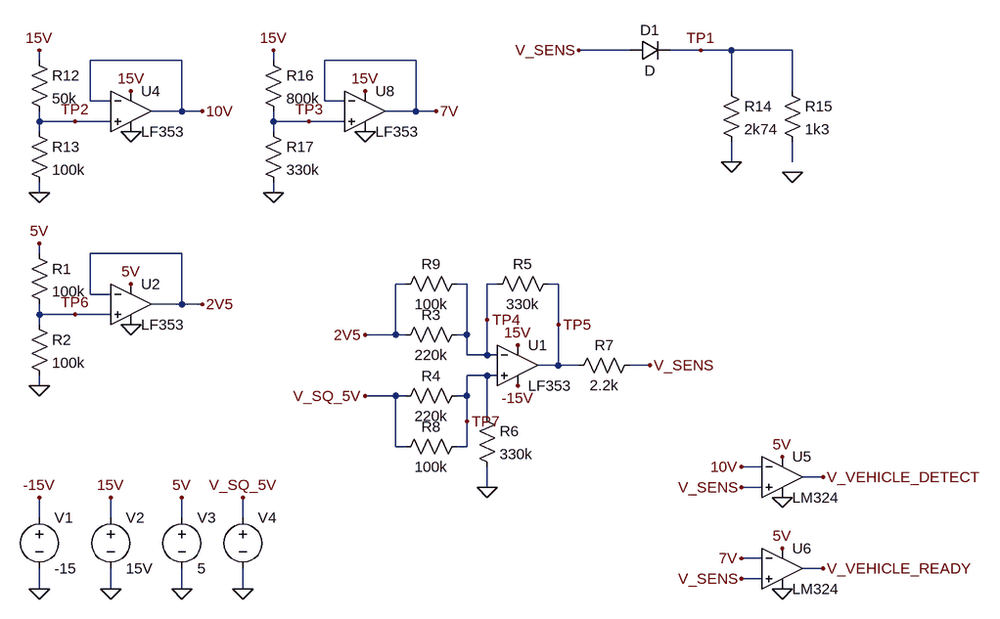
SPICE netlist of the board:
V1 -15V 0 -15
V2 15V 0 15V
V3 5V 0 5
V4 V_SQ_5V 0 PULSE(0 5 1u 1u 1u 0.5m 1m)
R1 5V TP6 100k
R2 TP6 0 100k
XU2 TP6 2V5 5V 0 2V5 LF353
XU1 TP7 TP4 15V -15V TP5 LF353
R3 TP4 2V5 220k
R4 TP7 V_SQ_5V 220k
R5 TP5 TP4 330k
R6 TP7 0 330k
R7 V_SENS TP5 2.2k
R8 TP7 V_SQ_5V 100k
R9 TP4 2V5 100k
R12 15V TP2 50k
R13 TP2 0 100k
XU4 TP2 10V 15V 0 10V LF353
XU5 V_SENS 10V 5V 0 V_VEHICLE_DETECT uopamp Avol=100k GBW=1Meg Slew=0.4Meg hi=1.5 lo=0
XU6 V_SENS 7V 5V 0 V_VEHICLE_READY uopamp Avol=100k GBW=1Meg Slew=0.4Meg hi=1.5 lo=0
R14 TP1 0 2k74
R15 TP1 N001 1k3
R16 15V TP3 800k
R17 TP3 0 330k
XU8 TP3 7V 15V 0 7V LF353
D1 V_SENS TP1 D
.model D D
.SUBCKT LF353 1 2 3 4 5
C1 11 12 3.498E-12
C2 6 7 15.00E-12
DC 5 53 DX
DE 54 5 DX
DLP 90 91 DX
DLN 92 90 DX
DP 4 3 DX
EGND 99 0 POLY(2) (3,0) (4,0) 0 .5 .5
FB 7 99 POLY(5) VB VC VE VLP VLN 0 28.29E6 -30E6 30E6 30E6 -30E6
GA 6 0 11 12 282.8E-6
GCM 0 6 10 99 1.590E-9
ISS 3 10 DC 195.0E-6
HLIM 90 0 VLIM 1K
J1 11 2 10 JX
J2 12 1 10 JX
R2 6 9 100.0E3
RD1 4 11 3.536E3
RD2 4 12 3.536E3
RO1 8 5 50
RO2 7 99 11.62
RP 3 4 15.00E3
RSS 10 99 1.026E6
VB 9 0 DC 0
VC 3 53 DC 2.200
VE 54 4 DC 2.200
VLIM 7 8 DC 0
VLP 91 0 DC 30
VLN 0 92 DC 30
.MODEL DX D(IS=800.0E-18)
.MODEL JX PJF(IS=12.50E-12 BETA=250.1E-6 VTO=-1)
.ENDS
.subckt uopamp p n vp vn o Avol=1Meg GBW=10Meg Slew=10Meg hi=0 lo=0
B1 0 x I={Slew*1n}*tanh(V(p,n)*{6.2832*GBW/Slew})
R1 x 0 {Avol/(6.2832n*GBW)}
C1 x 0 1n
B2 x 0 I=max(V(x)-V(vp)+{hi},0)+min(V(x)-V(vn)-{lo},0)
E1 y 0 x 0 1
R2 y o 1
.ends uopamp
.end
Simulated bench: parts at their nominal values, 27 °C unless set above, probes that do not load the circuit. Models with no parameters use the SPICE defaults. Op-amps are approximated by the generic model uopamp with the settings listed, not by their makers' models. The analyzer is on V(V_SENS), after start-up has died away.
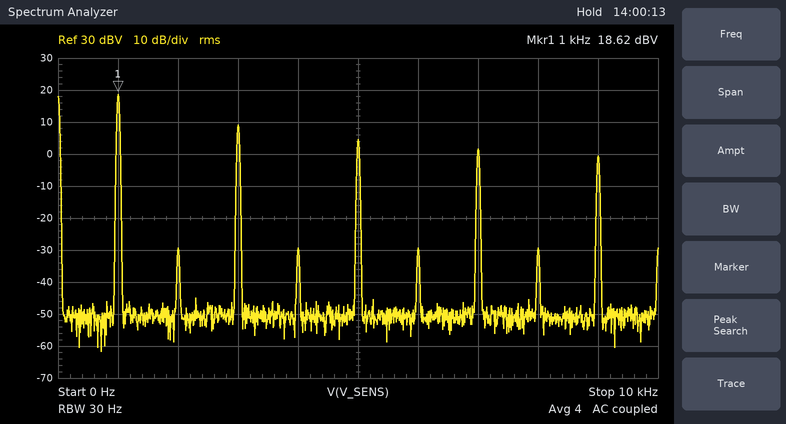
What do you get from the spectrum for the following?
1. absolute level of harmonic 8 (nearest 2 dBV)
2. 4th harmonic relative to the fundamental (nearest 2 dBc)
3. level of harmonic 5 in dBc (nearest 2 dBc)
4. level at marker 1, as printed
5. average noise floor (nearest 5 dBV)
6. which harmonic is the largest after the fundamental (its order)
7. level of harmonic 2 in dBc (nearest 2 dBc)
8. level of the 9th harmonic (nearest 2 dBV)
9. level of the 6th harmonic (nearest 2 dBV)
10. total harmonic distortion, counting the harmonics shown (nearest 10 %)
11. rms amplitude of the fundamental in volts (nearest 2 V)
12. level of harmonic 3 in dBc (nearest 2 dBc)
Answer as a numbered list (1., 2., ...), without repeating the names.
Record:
1. -30 dBV
2. -48 dBc
3. -14 dBc
4. 18.62 dBV
5. -50 dBV
6. 3
7. -48 dBc
8. 0 dBV
9. -30 dBV
10. 40 %
11. 8 V
12. -10 dBc
